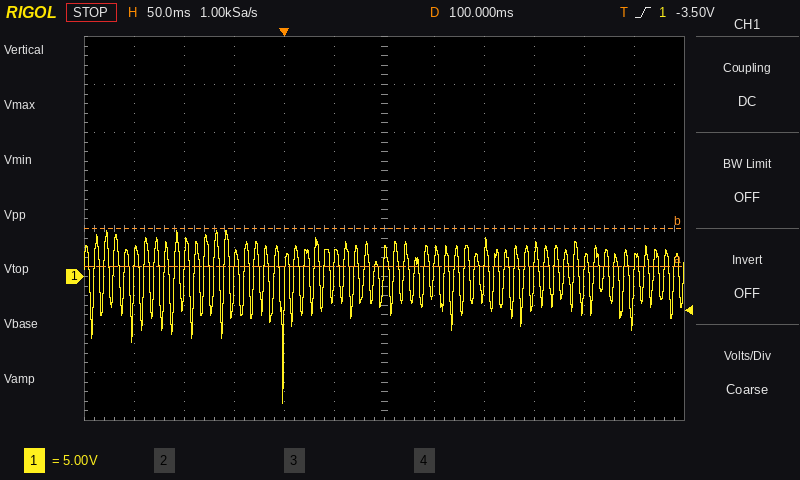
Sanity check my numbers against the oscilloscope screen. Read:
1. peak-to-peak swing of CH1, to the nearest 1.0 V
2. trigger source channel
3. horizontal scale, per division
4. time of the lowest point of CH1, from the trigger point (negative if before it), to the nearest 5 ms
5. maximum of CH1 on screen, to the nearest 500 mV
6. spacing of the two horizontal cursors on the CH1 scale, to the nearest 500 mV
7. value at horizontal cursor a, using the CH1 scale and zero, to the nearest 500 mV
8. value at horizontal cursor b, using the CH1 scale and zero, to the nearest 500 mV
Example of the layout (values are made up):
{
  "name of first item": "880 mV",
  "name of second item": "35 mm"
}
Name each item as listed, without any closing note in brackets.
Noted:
{
  "peak-to-peak swing of CH1, to the nearest 1.0 V": "18.0 V",
  "trigger source channel": "CH1",
  "horizontal scale, per division": "50 ms",
  "time of the lowest point of CH1, from the trigger point (negative if before it), to the nearest 5 ms": "0 ms",
  "maximum of CH1 on screen, to the nearest 500 mV": "5.0 V",
  "spacing of the two horizontal cursors on the CH1 scale, to the nearest 500 mV": "4.0 V",
  "value at horizontal cursor a, using the CH1 scale and zero, to the nearest 500 mV": "1.0 V",
  "value at horizontal cursor b, using the CH1 scale and zero, to the nearest 500 mV": "5.0 V"
}
